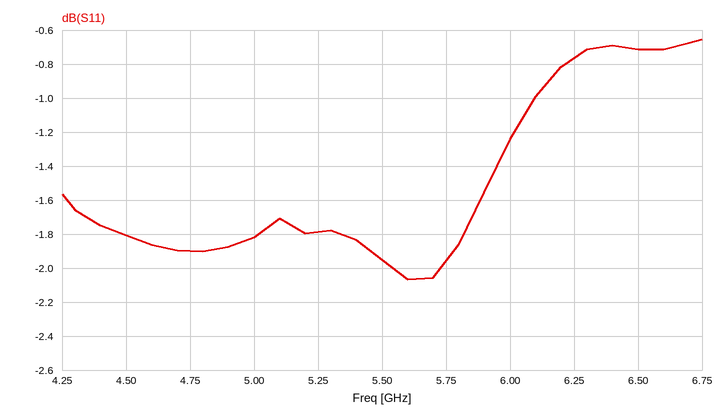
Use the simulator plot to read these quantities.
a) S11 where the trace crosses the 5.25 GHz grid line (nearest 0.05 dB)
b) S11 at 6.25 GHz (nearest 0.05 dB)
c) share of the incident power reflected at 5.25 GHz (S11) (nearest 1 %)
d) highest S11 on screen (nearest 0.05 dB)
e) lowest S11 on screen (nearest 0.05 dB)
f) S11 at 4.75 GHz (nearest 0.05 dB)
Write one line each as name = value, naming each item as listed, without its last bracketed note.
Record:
S11 where the trace crosses the 5.25 GHz grid line = -1.80 dB
S11 at 6.25 GHz = -0.75 dB
share of the incident power reflected at 5.25 GHz (S11) = 66 %
highest S11 on screen = -0.65 dB
lowest S11 on screen = -2.05 dB
S11 at 4.75 GHz = -1.90 dB
